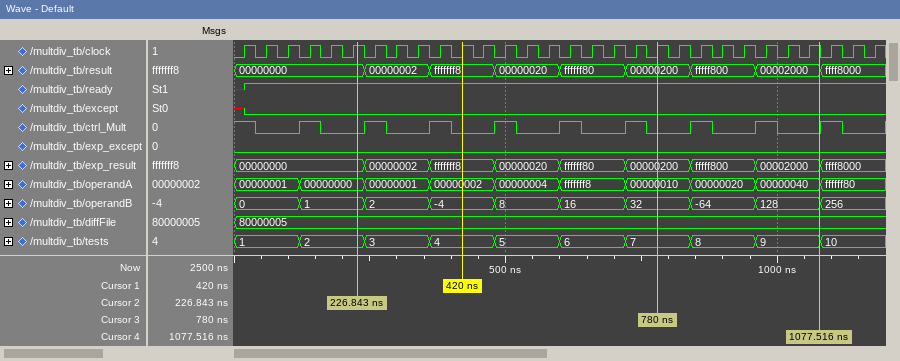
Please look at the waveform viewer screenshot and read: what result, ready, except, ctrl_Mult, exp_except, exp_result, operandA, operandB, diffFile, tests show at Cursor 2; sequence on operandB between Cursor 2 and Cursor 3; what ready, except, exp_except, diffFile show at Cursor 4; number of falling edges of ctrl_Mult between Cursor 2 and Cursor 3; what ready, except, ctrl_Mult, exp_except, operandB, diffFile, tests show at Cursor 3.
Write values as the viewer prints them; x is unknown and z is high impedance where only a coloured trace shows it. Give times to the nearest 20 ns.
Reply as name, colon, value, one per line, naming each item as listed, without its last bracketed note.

what result, ready, except, ctrl_Mult, exp_except, exp_result, operandA, operandB, diffFile, tests show at Cursor 2: result=00000000, ready=1, except=0, ctrl_Mult=0, exp_except=0, exp_result=00000000, operandA=00000000, operandB=1, diffFile=80000005, tests=2
sequence on operandB between Cursor 2 and Cursor 3: 1, 2, -4, 8, 16, 32
what ready, except, exp_except, diffFile show at Cursor 4: ready=1, except=0, exp_except=0, diffFile=80000005
number of falling edges of ctrl_Mult between Cursor 2 and Cursor 3: 5
what ready, except, ctrl_Mult, exp_except, operandB, diffFile, tests show at Cursor 3: ready=1, except=0, ctrl_Mult=0, exp_except=0, operandB=32, diffFile=80000005, tests=7
